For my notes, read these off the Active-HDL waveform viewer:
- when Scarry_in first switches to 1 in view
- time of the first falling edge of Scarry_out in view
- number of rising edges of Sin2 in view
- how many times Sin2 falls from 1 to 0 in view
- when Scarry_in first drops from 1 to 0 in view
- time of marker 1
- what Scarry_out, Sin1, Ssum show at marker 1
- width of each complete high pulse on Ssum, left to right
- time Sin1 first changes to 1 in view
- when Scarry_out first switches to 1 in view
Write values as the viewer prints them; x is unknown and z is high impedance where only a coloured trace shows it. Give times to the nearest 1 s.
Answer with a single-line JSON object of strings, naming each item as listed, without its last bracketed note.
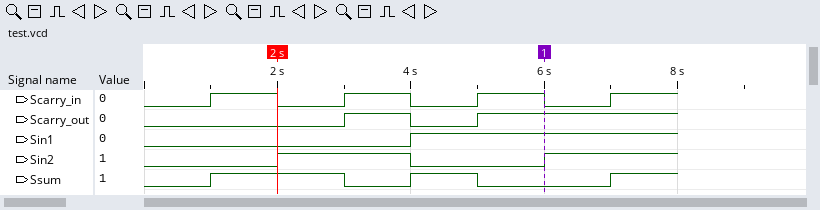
{"when Scarry_in first switches to 1 in view": "1 s", "time of the first falling edge of Scarry_out in view": "4 s", "number of rising edges of Sin2 in view": "2", "how many times Sin2 falls from 1 to 0 in view": "1", "when Scarry_in first drops from 1 to 0 in view": "2 s", "time of marker 1": "6 s", "what Scarry_out, Sin1, Ssum show at marker 1": "Scarry_out=1, Sin1=1, Ssum=0", "width of each complete high pulse on Ssum, left to right": "2 s, 1 s", "time Sin1 first changes to 1 in view": "4 s", "when Scarry_out first switches to 1 in view": "3 s"}
